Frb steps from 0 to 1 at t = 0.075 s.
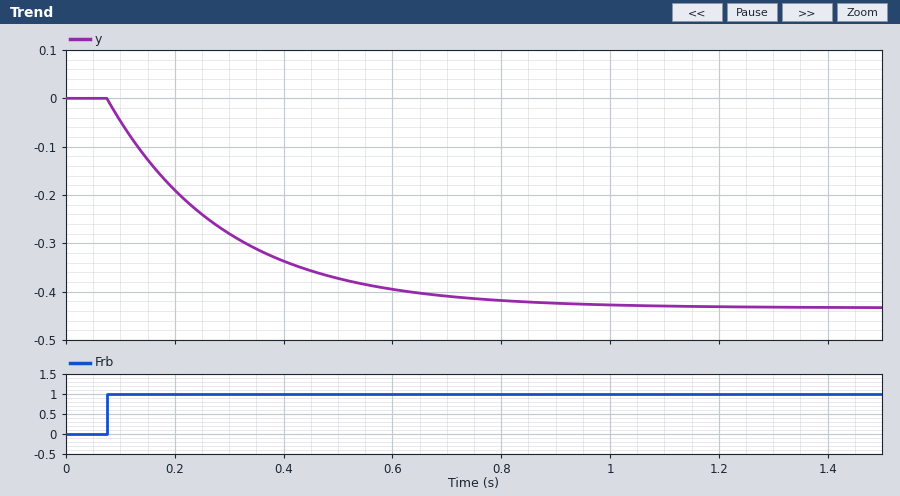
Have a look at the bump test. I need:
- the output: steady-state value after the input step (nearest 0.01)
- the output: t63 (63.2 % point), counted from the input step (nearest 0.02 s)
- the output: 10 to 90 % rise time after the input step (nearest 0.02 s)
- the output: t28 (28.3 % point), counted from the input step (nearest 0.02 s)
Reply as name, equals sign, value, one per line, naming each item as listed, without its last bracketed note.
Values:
the output: steady-state value after the input step = -0.43
the output: t63 (63.2 % point), counted from the input step = 0.22 s
the output: 10 to 90 % rise time after the input step = 0.48 s
the output: t28 (28.3 % point), counted from the input step = 0.08 s
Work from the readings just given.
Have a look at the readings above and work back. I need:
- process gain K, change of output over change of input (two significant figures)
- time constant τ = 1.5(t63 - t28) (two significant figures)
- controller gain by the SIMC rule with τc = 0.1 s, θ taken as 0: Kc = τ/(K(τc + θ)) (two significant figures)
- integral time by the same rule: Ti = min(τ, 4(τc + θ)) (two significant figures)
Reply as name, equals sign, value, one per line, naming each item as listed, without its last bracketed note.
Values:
process gain K, change of output over change of input = -0.43
time constant τ = 1.5(t63 - t28) = 0.21 s
controller gain by the SIMC rule with τc = 0.1 s, θ taken as 0: Kc = τ/(K(τc + θ)) = -4.9
integral time by the same rule: Ti = min(τ, 4(τc + θ)) = 0.21 s
